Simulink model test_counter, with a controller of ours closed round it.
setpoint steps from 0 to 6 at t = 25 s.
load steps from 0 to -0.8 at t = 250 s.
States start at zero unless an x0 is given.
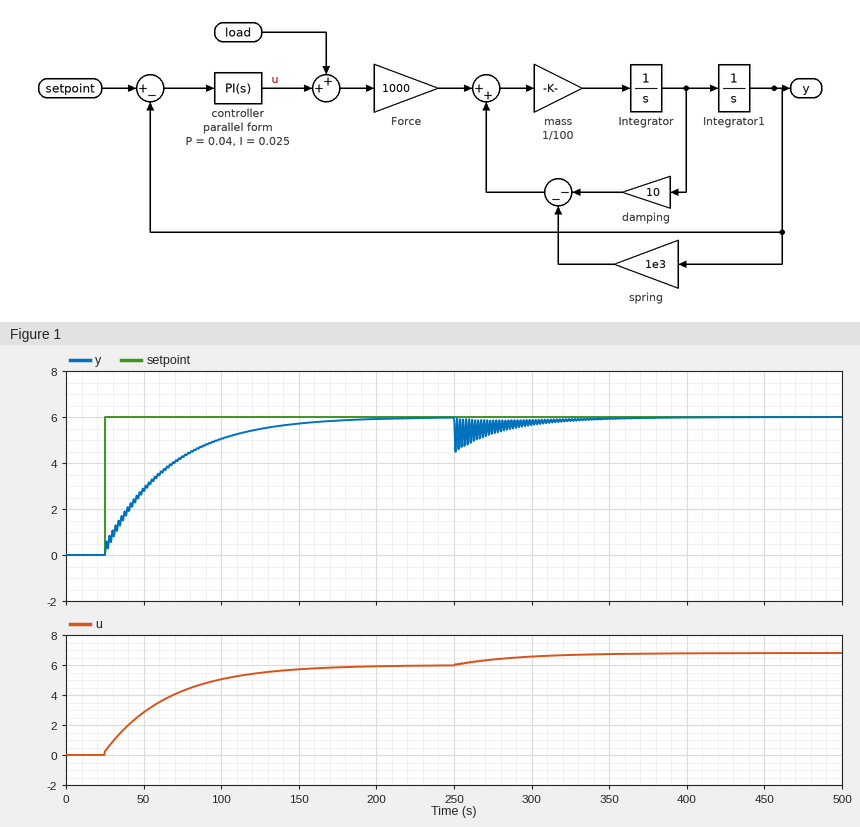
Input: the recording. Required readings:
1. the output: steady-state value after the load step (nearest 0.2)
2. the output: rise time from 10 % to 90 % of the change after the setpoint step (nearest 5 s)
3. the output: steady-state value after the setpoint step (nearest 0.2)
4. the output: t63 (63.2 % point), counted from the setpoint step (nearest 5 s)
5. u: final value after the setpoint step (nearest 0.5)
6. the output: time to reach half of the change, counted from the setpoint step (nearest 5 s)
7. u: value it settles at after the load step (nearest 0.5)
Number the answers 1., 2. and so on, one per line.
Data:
1. 6.0
2. 90 s
3. 6.0
4. 40 s
5. 6.0
6. 25 s
7. 7.0
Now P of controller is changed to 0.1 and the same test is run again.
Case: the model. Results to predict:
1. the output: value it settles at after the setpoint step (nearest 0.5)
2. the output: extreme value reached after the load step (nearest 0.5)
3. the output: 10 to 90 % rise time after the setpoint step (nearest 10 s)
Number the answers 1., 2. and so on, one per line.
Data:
1. 6.0
2. 4.5
3. 100 s
